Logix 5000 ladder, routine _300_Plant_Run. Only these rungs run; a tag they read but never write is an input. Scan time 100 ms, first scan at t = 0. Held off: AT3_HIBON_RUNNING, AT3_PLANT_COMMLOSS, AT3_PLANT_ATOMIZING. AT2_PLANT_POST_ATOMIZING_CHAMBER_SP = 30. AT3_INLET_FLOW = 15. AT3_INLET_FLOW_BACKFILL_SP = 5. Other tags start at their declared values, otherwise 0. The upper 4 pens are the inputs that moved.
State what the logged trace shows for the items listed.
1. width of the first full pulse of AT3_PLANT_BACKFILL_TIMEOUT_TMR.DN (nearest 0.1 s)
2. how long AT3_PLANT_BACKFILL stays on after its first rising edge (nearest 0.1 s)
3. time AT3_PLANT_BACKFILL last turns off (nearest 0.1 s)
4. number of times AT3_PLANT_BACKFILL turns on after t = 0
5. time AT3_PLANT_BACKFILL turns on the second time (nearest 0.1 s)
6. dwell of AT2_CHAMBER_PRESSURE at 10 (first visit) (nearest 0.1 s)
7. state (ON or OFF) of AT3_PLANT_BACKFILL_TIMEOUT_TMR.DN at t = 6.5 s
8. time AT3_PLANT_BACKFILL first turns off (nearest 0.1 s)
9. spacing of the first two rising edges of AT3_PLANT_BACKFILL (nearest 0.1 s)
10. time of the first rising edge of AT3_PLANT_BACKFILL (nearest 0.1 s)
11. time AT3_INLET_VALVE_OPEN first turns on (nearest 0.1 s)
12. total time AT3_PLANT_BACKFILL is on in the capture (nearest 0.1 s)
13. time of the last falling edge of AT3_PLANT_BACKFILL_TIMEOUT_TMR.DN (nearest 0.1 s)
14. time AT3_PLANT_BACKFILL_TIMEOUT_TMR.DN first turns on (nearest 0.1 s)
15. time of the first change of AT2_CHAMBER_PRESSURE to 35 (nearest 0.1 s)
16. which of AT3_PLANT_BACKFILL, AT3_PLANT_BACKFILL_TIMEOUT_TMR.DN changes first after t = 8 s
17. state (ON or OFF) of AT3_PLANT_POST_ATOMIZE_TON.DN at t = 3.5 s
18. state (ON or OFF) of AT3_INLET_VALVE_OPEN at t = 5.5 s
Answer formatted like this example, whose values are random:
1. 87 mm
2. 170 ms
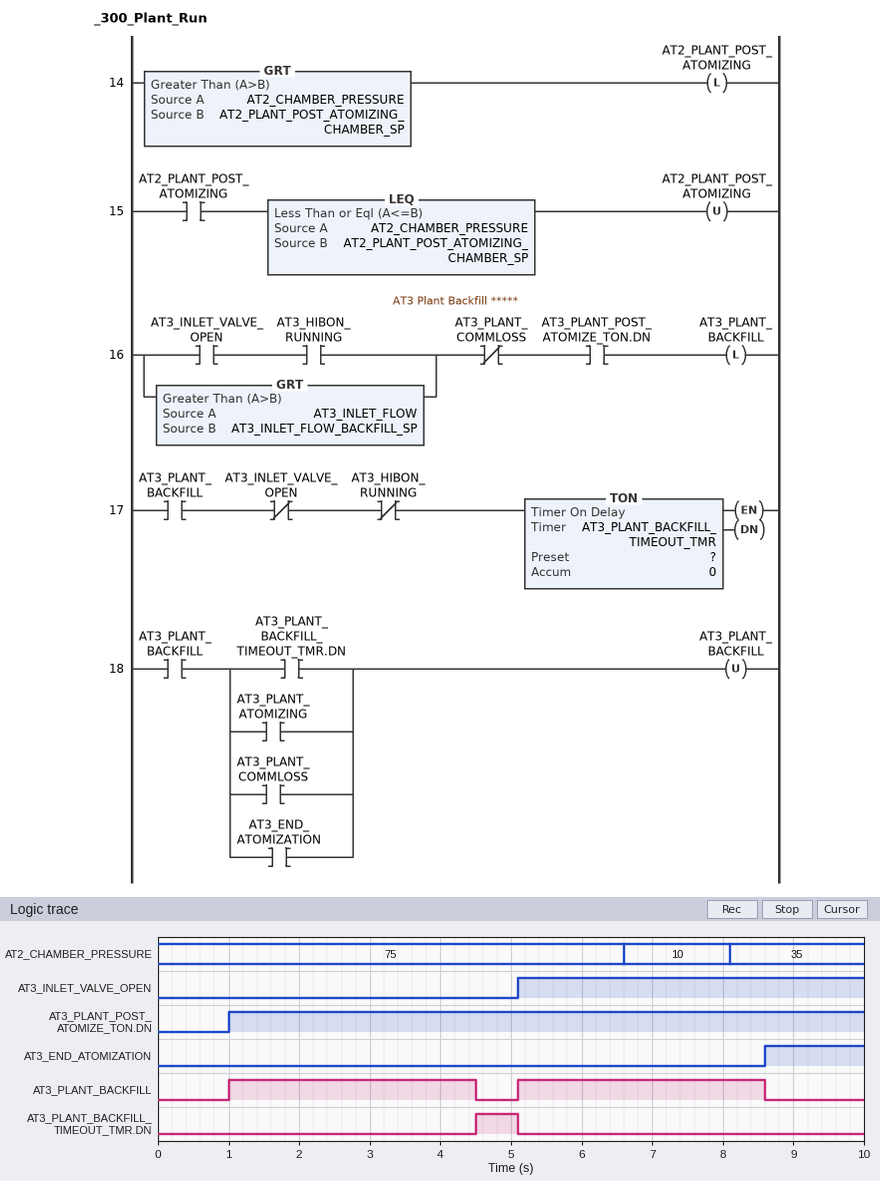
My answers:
1. 0.6 s
2. 3.5 s
3. 8.6 s
4. 2
5. 5.1 s
6. 1.5 s
7. OFF
8. 4.5 s
9. 4.1 s
10. 1.0 s
11. 5.1 s
12. 7.0 s
13. 5.1 s
14. 4.5 s
15. 8.1 s
16. AT3_PLANT_BACKFILL
17. ON
18. ON
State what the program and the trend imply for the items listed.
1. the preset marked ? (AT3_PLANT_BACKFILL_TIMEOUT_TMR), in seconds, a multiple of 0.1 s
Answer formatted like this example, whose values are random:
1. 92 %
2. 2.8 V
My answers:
1. 3.5 s
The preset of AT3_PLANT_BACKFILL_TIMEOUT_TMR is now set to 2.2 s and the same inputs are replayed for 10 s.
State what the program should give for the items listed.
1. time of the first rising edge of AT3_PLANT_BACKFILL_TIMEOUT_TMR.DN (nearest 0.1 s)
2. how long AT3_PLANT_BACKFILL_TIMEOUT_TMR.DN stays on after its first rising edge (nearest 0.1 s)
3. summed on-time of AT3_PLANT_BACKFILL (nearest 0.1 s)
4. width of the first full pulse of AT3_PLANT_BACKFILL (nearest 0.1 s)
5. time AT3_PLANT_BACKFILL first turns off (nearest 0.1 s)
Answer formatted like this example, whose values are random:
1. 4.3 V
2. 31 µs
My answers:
1. 3.2 s
2. 1.9 s
3. 5.7 s
4. 2.2 s
5. 3.2 s
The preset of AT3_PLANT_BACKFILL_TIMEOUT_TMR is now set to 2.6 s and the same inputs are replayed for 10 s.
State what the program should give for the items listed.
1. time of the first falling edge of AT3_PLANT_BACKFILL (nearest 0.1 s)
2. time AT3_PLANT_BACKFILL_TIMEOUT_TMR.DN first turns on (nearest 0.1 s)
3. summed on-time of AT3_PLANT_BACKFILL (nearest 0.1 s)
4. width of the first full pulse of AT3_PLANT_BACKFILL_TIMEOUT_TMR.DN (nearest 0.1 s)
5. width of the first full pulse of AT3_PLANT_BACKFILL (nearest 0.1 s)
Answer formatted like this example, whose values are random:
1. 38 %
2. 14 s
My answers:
1. 3.6 s
2. 3.6 s
3. 6.1 s
4. 1.5 s
5. 2.6 s
